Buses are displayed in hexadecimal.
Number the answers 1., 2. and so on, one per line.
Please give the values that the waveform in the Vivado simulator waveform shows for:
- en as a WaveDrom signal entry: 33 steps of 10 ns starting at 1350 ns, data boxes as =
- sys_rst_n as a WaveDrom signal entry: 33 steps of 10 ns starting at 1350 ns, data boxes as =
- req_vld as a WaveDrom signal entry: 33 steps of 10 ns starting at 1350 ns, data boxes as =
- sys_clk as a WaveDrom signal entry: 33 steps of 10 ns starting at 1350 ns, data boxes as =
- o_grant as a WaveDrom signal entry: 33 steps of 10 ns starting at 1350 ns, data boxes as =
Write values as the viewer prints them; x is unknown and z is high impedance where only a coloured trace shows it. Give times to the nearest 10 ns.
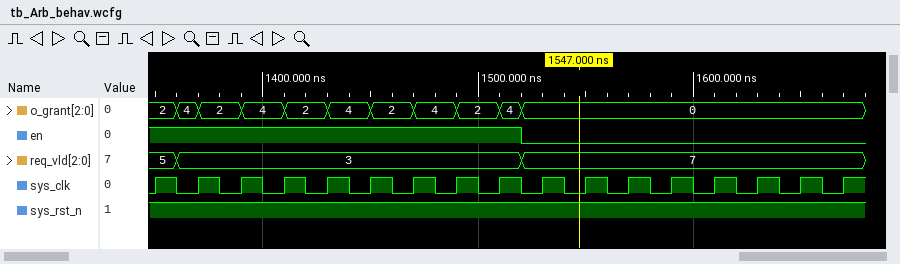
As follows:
1. {name: 'en', wave: '1................0...............'}
2. {name: 'sys_rst_n', wave: '1................................'}
3. {name: 'req_vld', wave: '==...............=...............', data: '5 3 7'}
4. {name: 'sys_clk', wave: '101010101010101010101010101010101'}
5. {name: 'o_grant', wave: '===.=.=.=.=.=.=.==...............', data: '2 4 2 4 2 4 2 4 2 4 0'}
